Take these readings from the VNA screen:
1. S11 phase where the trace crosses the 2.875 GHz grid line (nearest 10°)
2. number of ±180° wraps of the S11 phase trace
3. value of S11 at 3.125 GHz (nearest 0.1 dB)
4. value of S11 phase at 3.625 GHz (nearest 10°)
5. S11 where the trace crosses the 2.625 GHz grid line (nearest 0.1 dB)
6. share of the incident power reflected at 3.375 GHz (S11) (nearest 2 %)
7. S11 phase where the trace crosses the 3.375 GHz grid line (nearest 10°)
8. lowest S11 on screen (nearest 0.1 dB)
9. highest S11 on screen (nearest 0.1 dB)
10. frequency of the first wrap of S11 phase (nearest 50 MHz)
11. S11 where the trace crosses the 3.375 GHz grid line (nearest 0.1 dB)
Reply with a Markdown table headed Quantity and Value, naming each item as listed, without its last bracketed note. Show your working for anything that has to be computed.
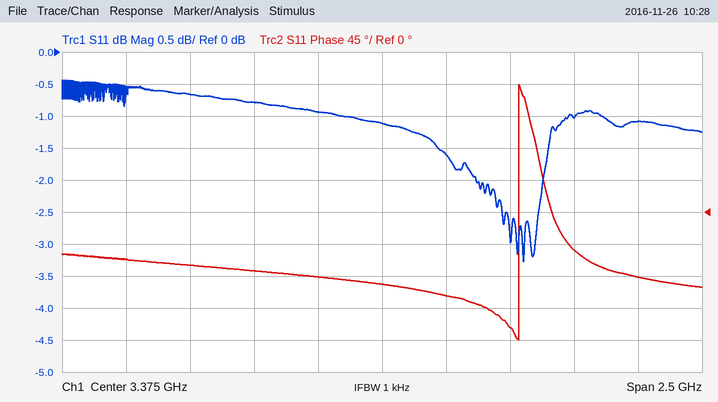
| Quantity | Value |
|---|---|
| S11 phase where the trace crosses the 2.875 GHz grid line | -80° |
| number of ±180° wraps of the S11 phase trace | 1 |
| value of S11 at 3.125 GHz | -0.9 dB |
| value of S11 phase at 3.625 GHz | -120° |
| S11 where the trace crosses the 2.625 GHz grid line | -0.7 dB |
| share of the incident power reflected at 3.375 GHz (S11) | 10^(-1.1/10) ≈ 78 % |
| S11 phase where the trace crosses the 3.375 GHz grid line | -100° |
| lowest S11 on screen | -3.3 dB |
| highest S11 on screen | -0.4 dB |
| frequency of the first wrap of S11 phase | 3.90 GHz |
| S11 where the trace crosses the 3.375 GHz grid line | -1.1 dB |
